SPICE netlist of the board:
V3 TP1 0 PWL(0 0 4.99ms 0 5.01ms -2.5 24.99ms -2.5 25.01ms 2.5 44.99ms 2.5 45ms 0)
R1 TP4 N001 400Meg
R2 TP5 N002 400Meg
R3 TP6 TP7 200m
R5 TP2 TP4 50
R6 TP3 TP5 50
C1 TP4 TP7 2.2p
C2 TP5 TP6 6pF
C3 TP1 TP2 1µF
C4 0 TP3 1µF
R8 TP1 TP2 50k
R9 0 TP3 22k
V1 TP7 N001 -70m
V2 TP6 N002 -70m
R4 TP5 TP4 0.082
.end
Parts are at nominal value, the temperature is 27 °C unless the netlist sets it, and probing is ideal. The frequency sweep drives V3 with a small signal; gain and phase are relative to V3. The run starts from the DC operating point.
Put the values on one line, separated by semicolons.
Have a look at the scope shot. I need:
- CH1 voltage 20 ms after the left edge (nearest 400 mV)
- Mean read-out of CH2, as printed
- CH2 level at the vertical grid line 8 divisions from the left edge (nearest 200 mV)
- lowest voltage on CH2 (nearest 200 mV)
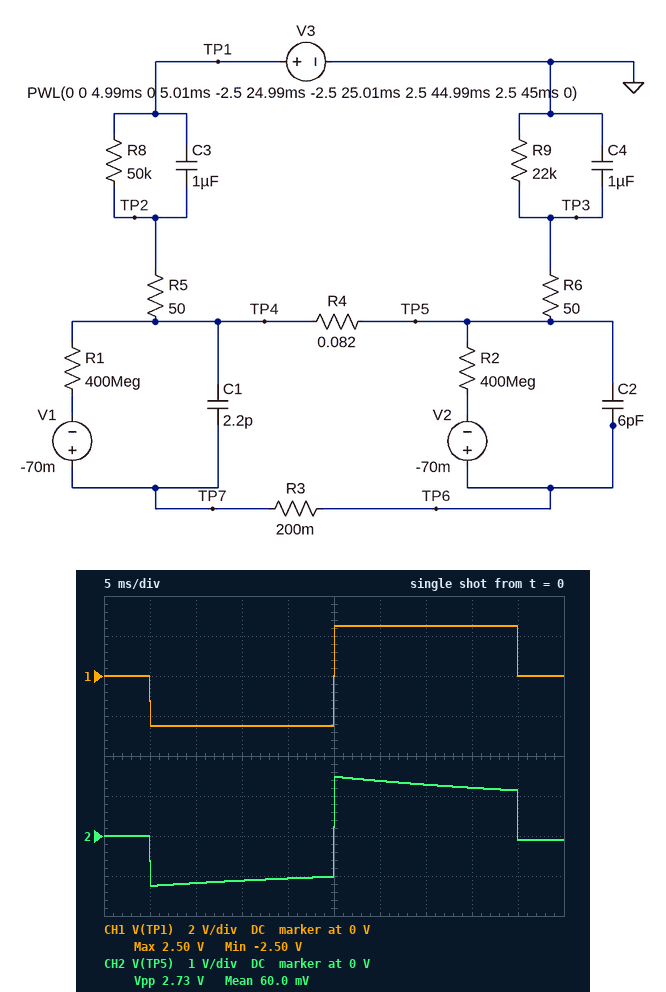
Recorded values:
-2.4 V; 60.0 mV; 1.2 V; -1.2 V
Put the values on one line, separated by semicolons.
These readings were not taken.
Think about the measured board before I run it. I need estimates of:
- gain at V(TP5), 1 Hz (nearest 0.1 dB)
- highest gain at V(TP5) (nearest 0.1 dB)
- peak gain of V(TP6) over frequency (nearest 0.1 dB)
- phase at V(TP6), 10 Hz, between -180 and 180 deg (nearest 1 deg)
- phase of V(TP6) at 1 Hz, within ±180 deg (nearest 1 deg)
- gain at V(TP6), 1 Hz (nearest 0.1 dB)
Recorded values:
-10.0 dB; -6.0 dB; -6.0 dB; 10 deg; 7 deg; -10.0 dB
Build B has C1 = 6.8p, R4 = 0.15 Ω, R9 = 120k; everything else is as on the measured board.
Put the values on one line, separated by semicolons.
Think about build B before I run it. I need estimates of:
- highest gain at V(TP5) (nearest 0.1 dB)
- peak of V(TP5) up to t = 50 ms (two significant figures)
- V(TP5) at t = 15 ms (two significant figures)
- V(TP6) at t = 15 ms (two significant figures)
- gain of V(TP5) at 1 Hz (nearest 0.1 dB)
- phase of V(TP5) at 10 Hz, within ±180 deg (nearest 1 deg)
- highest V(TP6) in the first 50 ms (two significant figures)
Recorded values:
-3.0 dB; 1.3 V; -1.3 V; -1.4 V; -3.4 dB; -5 deg; 1.2 V
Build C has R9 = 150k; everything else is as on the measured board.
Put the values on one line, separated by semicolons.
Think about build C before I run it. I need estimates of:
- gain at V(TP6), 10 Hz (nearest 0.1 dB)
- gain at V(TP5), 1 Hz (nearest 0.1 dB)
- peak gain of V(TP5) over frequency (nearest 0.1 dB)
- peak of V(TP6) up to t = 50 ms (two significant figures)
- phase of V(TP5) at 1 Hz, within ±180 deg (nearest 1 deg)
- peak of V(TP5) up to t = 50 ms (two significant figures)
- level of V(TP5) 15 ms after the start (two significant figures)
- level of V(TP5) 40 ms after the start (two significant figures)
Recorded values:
-5.8 dB; -3.0 dB; -2.5 dB; 1.2 V; -8 deg; 1.3 V; -1.3 V; 1.2 V
